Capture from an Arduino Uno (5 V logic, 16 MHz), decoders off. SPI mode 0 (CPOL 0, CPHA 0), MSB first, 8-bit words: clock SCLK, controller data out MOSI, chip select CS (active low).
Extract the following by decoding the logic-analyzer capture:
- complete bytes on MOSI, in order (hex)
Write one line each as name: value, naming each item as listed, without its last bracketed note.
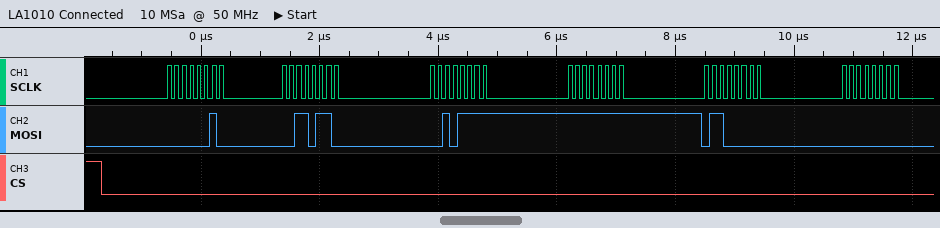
complete bytes on MOSI, in order: 02 36 2F FF 60 00
